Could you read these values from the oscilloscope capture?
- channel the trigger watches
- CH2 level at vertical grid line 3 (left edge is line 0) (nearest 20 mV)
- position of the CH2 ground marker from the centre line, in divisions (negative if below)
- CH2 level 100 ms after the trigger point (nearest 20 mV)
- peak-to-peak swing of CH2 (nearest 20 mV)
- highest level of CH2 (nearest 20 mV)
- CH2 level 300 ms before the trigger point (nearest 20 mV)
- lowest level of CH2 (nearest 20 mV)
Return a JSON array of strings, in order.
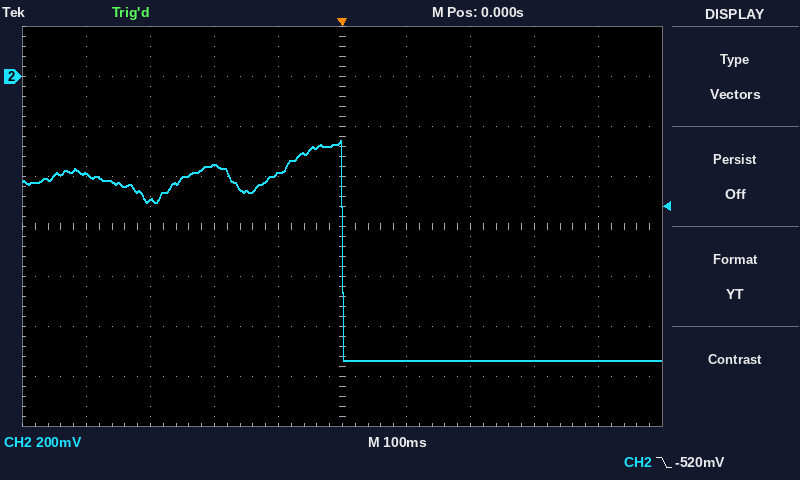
["CH2", "-360 mV", "+3.0 div", "-1.14 V", "880 mV", "-260 mV", "-500 mV", "-1.14 V"]
